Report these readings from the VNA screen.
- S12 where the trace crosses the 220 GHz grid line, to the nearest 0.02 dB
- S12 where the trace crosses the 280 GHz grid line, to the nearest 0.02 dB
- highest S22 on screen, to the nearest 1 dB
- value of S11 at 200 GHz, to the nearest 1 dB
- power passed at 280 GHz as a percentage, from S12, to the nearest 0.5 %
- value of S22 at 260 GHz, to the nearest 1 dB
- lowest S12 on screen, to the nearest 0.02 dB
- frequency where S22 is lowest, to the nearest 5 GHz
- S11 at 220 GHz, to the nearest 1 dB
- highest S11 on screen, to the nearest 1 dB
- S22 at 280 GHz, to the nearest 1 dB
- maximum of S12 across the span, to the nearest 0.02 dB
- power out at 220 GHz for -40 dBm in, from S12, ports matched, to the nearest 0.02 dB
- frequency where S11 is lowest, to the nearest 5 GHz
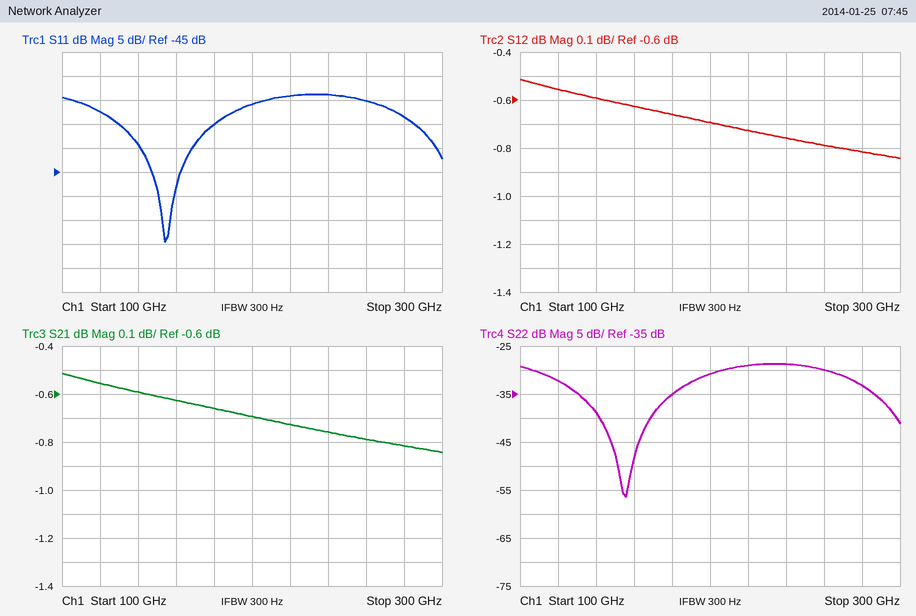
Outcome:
-0.72 dB
-0.82 dB
-29 dB
-31 dB
83.0 %
-30 dB
-0.84 dB
155 GHz
-29 dB
-29 dB
-33 dB
-0.52 dB
-40.72 dBm
155 GHz
